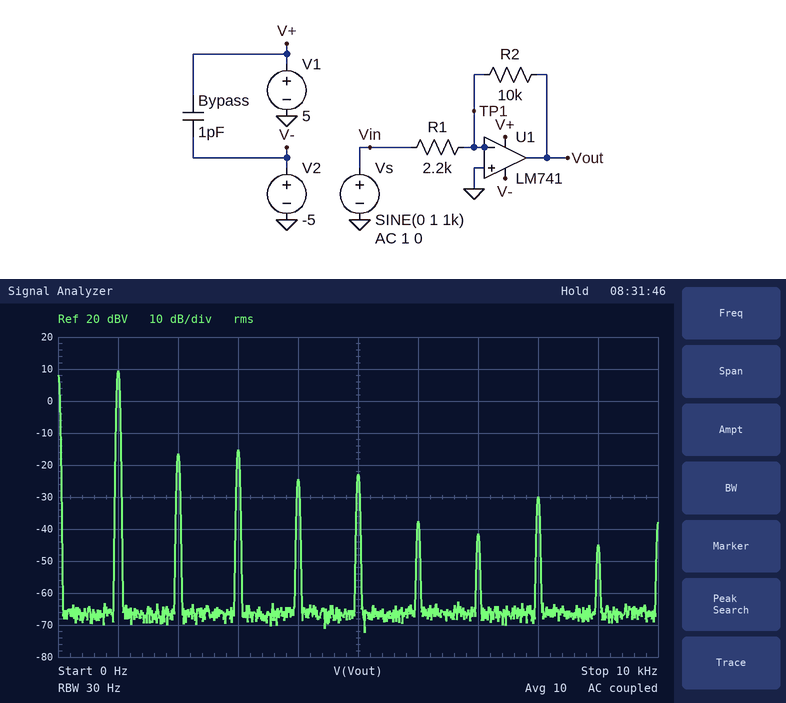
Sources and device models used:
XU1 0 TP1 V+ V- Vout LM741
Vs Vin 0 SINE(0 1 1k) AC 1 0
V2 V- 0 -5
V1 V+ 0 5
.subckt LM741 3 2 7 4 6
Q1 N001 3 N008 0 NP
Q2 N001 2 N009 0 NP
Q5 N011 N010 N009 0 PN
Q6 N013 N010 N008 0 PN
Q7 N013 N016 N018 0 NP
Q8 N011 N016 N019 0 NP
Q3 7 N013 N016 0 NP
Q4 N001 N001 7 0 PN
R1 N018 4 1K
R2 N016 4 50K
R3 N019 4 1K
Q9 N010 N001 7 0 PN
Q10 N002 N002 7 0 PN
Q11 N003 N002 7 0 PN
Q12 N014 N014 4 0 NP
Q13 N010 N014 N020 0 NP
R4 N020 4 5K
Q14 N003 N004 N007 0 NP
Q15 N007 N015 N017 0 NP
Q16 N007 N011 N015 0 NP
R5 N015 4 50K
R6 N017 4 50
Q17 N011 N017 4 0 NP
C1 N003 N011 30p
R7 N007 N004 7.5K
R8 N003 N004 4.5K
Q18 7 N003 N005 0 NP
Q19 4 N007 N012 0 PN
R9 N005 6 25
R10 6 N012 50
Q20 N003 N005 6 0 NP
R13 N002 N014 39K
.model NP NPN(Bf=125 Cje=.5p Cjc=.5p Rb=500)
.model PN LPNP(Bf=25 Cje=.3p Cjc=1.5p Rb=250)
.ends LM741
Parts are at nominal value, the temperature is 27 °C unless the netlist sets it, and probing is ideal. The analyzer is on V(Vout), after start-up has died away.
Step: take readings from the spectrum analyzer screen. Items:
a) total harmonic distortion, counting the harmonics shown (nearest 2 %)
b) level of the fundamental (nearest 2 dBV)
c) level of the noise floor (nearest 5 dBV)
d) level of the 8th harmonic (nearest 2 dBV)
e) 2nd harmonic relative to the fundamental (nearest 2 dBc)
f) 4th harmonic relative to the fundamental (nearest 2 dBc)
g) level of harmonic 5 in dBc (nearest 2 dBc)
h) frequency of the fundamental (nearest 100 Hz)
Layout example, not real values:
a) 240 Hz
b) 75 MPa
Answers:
a) 8 %
b) 10 dBV
c) -65 dBV
d) -30 dBV
e) -26 dBc
f) -34 dBc
g) -32 dBc
h) 1.0 kHz
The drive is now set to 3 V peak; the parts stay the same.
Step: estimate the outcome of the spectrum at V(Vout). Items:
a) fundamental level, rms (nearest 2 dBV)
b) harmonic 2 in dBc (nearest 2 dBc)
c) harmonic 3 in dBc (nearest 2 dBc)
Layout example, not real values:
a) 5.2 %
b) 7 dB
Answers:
a) 10 dBV
b) -32 dBc
c) -10 dBc
